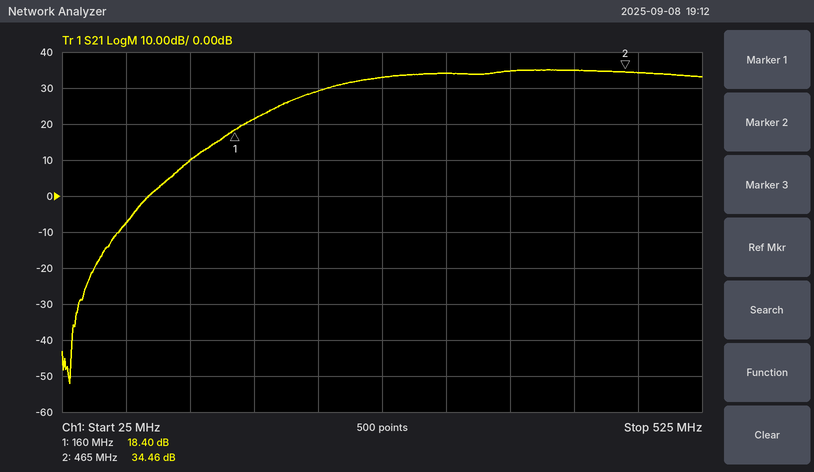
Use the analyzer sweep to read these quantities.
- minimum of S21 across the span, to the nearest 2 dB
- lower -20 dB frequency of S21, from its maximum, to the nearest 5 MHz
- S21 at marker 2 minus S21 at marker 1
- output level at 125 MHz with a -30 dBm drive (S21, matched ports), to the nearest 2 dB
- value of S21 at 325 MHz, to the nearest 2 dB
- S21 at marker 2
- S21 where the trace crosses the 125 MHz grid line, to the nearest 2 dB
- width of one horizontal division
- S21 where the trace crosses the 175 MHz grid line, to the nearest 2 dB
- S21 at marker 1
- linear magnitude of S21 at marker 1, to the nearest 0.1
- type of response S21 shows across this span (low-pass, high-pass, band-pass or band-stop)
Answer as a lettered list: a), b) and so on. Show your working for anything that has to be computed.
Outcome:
a) -52 dB
b) 145 MHz
c) 34.46 − (18.4) = 16.06 dB
d) -30 dBm + (10 dB) = -20 dBm
e) 34 dB
f) 34.46 dB
g) 10 dB
h) 50 MHz
i) 22 dB
j) 18.40 dB
k) 10^(18.4/20) ≈ 8.3
l) high-pass
